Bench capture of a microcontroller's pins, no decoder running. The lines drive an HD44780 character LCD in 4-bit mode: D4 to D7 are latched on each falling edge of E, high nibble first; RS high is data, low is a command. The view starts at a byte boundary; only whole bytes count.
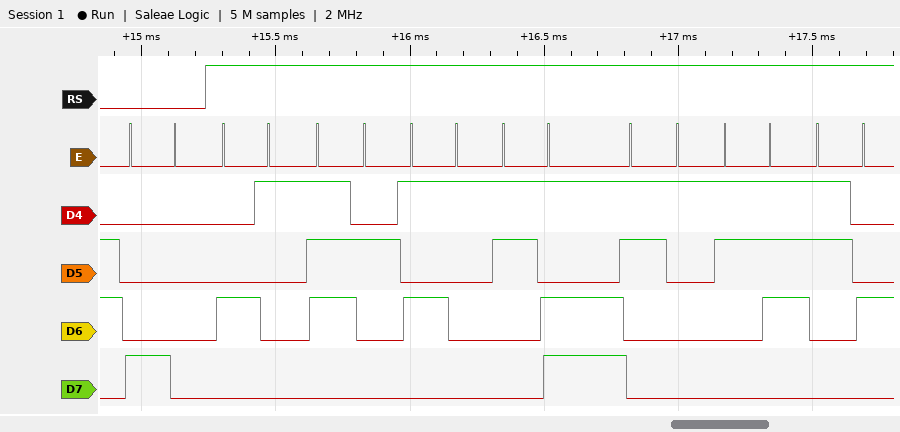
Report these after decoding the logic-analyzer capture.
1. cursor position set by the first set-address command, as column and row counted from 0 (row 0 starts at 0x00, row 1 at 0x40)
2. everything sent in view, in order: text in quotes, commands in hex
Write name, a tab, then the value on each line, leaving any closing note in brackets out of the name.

cursor position set by the first set-address command, as column and row counted from 0	column 0, row 0
everything sent in view, in order: text in quotes, commands in hex	0x80 "ArQ=174"
